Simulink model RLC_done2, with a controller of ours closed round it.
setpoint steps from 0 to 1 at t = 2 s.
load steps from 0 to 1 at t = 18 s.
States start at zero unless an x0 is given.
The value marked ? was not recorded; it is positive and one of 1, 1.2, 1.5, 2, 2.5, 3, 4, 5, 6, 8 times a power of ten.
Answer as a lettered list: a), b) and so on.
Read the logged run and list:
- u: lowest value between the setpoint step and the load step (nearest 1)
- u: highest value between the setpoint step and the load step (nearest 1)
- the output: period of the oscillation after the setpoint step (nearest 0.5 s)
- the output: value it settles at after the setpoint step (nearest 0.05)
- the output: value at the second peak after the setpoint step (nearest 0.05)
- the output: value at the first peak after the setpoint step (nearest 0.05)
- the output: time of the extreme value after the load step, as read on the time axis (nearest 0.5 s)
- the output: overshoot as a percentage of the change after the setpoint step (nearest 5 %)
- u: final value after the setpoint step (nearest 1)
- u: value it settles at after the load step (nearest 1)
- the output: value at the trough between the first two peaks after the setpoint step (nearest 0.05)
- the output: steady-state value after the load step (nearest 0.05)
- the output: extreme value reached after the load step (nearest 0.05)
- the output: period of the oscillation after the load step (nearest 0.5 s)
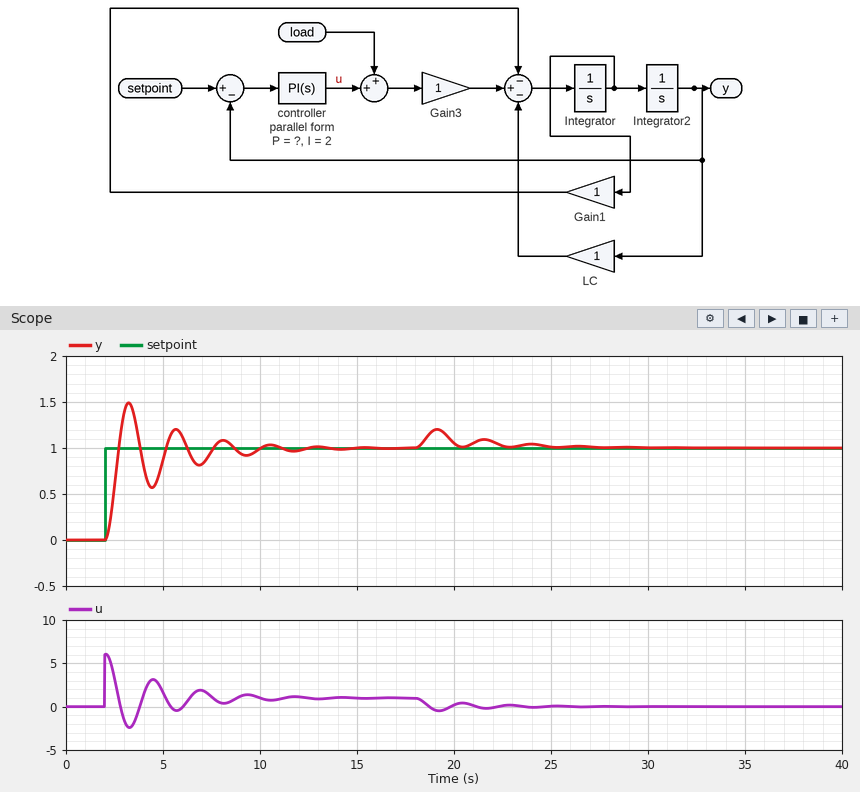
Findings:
a) -2
b) 6
c) 2.5 s
d) 1.00
e) 1.20
f) 1.50
g) 19.0 s
h) 50 %
i) 1
j) 0
k) 0.55
l) 1.00
m) 1.20
n) 2.5 s
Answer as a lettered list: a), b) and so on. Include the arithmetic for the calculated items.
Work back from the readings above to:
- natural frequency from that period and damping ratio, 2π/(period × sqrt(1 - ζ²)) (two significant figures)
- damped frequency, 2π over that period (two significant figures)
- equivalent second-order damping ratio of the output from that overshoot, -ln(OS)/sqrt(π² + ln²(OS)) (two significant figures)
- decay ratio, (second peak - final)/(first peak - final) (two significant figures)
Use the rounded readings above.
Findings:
a) 2π / (2.5 × sqrt(1 - 0.22²)) = 2.6 rad/s
b) 2π / 2.5 = 2.5 rad/s
c) ln(0.5) = -0.693; 0.693 / sqrt(9.870 + 0.480) = 0.22
d) (1.2 - 1) / (1.5 - 1) = 0.40
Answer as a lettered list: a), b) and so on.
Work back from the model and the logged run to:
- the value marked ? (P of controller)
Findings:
a) 6
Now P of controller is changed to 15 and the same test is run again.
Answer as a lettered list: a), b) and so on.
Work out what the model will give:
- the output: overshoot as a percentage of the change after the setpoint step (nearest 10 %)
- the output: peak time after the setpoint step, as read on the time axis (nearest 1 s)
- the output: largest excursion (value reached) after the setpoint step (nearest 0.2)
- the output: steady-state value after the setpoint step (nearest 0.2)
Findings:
a) 60 %
b) 3 s
c) 1.6
d) 1.0
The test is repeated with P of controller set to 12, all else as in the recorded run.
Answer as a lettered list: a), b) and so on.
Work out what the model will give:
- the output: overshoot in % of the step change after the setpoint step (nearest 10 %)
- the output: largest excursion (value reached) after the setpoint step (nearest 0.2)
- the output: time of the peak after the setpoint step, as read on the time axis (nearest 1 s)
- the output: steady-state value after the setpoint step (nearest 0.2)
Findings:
a) 60 %
b) 1.6
c) 3 s
d) 1.0
